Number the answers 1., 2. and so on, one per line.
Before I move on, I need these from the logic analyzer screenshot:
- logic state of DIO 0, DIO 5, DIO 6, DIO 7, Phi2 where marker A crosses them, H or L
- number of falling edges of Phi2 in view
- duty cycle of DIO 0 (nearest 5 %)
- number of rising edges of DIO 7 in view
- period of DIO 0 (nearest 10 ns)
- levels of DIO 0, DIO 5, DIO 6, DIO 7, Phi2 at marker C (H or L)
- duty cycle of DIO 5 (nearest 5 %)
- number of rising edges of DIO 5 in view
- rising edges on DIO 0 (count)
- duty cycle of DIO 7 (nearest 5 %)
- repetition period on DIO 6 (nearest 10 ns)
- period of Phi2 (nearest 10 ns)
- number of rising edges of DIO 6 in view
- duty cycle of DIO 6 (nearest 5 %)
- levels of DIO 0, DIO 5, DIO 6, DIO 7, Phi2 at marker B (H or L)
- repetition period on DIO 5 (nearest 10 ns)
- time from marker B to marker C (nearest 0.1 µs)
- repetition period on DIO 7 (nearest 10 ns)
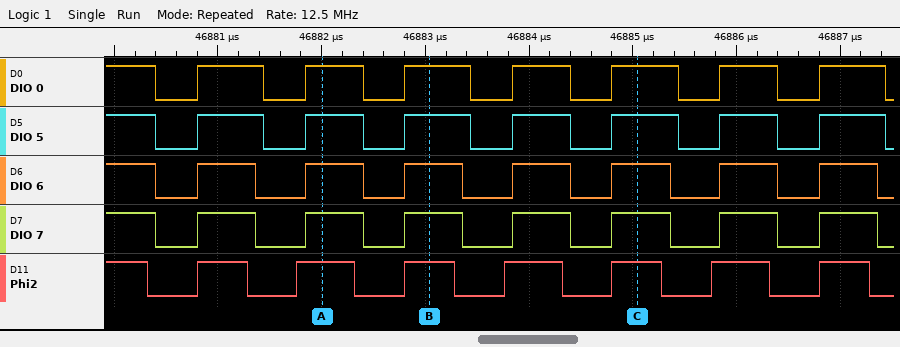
1. DIO 0=H, DIO 5=H, DIO 6=H, DIO 7=H, Phi2=H
2. 8
3. 60 %
4. 7
5. 1000 ns
6. DIO 0=H, DIO 5=H, DIO 6=H, DIO 7=H, Phi2=H
7. 60 %
8. 7
9. 7
10. 55 %
11. 1000 ns
12. 1000 ns
13. 7
14. 55 %
15. DIO 0=H, DIO 5=H, DIO 6=H, DIO 7=H, Phi2=H
16. 1000 ns
17. 2 µs
18. 1000 ns
